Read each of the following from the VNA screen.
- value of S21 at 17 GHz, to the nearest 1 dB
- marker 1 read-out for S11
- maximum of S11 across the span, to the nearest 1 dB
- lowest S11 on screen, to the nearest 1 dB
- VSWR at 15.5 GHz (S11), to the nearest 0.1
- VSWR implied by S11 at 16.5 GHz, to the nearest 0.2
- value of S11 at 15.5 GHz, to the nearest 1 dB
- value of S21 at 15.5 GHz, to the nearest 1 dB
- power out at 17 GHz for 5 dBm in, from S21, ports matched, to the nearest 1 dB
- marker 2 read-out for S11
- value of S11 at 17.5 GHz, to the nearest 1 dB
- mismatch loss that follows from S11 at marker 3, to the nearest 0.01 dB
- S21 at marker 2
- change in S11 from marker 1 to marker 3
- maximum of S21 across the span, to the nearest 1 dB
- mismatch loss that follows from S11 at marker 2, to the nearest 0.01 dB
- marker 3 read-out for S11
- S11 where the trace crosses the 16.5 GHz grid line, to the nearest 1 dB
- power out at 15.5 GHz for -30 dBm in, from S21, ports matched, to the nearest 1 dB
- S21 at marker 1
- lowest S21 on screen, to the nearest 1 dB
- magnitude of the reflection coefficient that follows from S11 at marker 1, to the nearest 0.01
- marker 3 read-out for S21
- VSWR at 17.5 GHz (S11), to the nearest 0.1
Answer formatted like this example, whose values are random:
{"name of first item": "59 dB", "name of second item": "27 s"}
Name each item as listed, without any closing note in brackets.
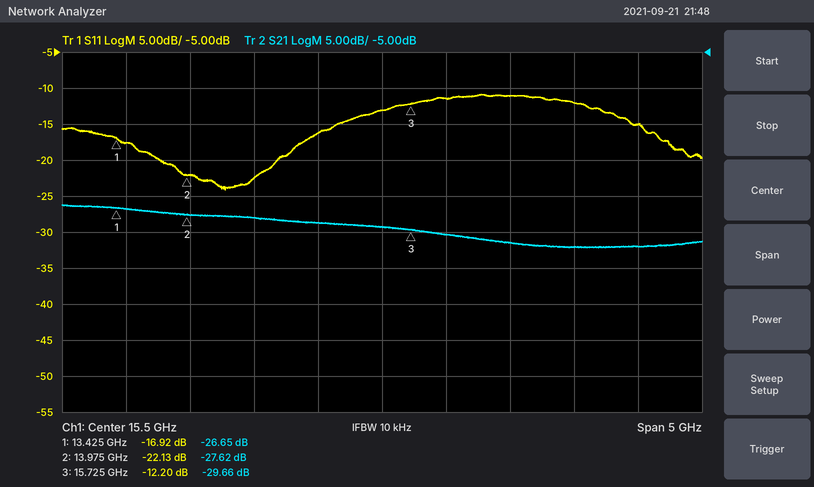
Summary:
{"value of S21 at 17 GHz, to the nearest 1 dB": "-32 dB", "marker 1 read-out for S11": "-16.92 dB", "maximum of S11 across the span, to the nearest 1 dB": "-11 dB", "lowest S11 on screen, to the nearest 1 dB": "-24 dB", "VSWR at 15.5 GHz (S11), to the nearest 0.1": "1.6", "VSWR implied by S11 at 16.5 GHz, to the nearest 0.2": "1.8", "value of S11 at 15.5 GHz, to the nearest 1 dB": "-13 dB", "value of S21 at 15.5 GHz, to the nearest 1 dB": "-29 dB", "power out at 17 GHz for 5 dBm in, from S21, ports matched, to the nearest 1 dB": "-27 dBm", "marker 2 read-out for S11": "-22.13 dB", "value of S11 at 17.5 GHz, to the nearest 1 dB": "-15 dB", "mismatch loss that follows from S11 at marker 3, to the nearest 0.01 dB": "0.27 dB", "S21 at marker 2": "-27.62 dB", "change in S11 from marker 1 to marker 3": "4.72 dB", "maximum of S21 across the span, to the nearest 1 dB": "-26 dB", "mismatch loss that follows from S11 at marker 2, to the nearest 0.01 dB": "0.03 dB", "marker 3 read-out for S11": "-12.20 dB", "S11 where the trace crosses the 16.5 GHz grid line, to the nearest 1 dB": "-11 dB", "power out at 15.5 GHz for -30 dBm in, from S21, ports matched, to the nearest 1 dB": "-59 dBm", "S21 at marker 1": "-26.65 dB", "lowest S21 on screen, to the nearest 1 dB": "-32 dB", "magnitude of the reflection coefficient that follows from S11 at marker 1, to the nearest 0.01": "0.14", "marker 3 read-out for S21": "-29.66 dB", "VSWR at 17.5 GHz (S11), to the nearest 0.1": "1.4"}
